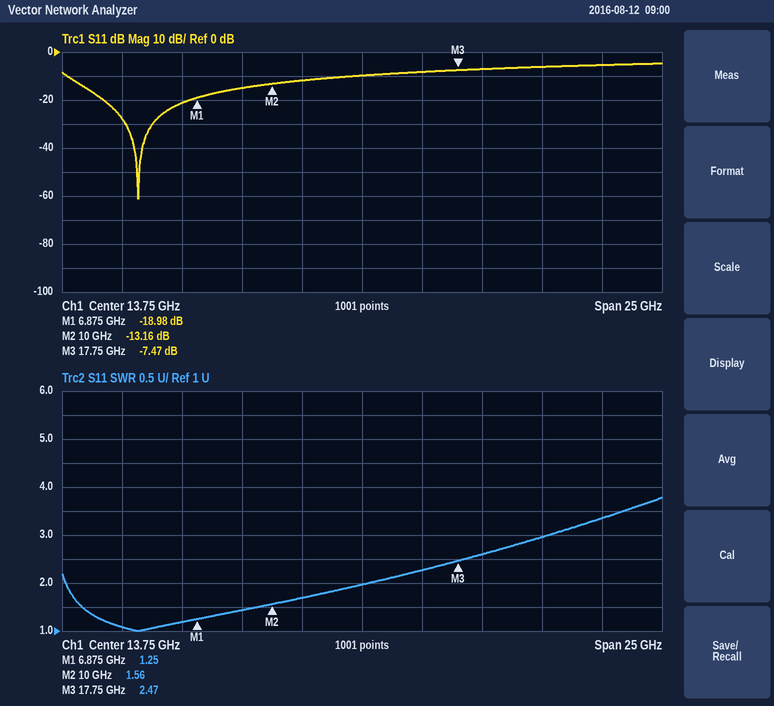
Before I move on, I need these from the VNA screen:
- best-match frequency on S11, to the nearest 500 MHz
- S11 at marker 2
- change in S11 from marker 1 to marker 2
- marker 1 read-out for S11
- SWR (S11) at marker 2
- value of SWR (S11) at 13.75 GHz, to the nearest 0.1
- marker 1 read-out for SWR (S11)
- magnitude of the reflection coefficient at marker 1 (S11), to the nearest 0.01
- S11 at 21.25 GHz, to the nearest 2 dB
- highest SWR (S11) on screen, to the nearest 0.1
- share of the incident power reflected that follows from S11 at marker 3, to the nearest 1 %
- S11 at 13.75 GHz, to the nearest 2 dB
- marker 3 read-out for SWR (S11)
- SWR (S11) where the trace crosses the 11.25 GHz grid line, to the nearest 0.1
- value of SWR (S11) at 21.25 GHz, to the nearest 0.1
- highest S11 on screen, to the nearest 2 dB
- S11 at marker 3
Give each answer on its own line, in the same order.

4.5 GHz
-13.16 dB
5.82 dB
-18.98 dB
1.56
2.0
1.25
0.11
-6 dB
3.8
18 %
-10 dB
2.47
1.7
3.0
-4 dB
-7.47 dB
